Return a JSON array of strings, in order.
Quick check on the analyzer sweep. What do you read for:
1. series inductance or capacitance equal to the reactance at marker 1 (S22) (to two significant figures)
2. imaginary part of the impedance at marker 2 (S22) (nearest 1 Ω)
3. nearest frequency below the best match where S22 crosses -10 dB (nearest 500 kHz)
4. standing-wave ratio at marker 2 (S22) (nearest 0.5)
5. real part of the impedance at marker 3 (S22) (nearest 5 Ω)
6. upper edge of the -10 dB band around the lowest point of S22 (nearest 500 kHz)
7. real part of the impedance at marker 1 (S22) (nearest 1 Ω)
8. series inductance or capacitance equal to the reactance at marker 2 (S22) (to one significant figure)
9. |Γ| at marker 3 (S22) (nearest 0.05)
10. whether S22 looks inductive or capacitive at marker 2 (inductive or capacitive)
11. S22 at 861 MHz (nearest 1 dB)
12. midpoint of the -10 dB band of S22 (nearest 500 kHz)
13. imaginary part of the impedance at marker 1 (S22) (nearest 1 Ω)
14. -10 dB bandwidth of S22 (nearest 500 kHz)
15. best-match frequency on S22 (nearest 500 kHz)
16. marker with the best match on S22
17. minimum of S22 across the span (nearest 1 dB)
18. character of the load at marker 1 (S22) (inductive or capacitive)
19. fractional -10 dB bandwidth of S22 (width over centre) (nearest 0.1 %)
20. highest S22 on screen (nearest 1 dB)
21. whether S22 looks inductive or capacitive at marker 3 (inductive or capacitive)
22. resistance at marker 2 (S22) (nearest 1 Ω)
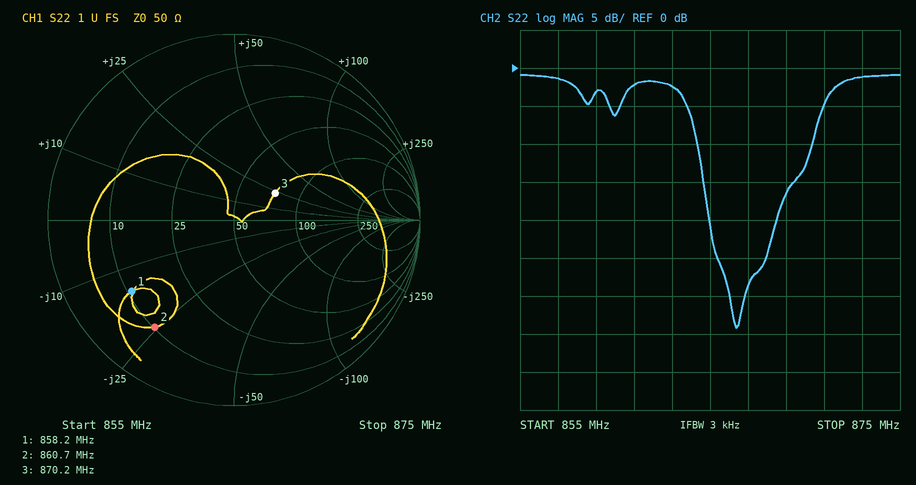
["12 pF", "-24 Ω", "864.5 MHz", "6.0", "75 Ω", "870.5 MHz", "11 Ω", "8 pF", "0.25", "capacitive", "-2 dB", "867.5 MHz", "-15 Ω", "6.0 MHz", "866.5 MHz", "marker 3", "-34 dB", "capacitive", "0.7 %", "-1 dB", "inductive", "10 Ω"]
